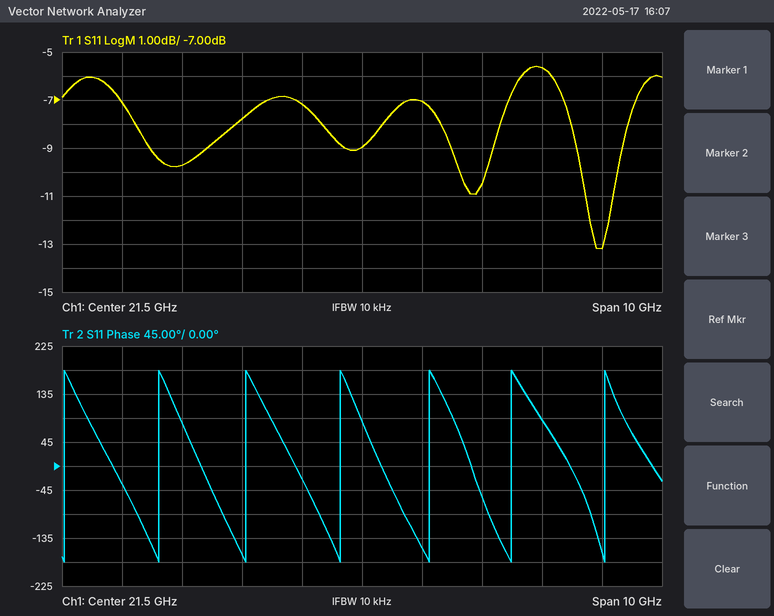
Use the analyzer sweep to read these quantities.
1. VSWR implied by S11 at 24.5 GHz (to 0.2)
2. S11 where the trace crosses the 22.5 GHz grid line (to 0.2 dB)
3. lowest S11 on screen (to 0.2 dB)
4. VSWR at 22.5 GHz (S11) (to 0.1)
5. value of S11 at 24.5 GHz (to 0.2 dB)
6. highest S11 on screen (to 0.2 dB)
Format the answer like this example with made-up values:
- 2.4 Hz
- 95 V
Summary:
- 3.2
- -7.0 dB
- -13.2 dB
- 2.6
- -5.6 dB
- -5.6 dB
